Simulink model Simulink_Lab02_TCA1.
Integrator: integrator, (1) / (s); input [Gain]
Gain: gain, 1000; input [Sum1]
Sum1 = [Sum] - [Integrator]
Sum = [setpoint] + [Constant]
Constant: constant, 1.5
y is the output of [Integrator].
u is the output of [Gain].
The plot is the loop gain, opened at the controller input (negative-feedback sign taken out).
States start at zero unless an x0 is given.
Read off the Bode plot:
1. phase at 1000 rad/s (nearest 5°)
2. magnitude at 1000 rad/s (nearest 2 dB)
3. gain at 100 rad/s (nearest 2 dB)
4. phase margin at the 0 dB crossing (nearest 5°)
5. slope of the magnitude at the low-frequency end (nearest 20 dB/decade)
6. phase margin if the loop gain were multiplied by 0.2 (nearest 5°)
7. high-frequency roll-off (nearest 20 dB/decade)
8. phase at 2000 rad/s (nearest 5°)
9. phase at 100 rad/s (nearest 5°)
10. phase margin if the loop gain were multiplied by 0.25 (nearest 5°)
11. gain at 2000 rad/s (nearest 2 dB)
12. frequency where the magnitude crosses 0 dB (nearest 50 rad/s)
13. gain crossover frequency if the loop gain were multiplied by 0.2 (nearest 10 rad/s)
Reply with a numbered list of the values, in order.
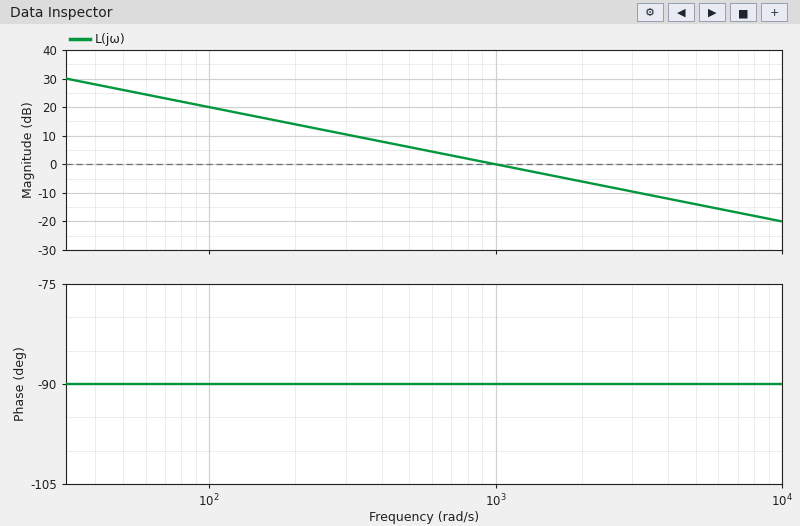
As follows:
1. -90°
2. 0 dB
3. 20 dB
4. 90°
5. -20 dB/decade
6. 90°
7. -20 dB/decade
8. -90°
9. -90°
10. 90°
11. -6 dB
12. 1000 rad/s
13. 200 rad/s
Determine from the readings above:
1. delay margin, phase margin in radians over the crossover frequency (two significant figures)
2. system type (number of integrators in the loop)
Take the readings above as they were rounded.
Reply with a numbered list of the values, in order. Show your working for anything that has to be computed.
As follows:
1. 90 × π / 180 / 1000 = 0.0016 s
2. 1
